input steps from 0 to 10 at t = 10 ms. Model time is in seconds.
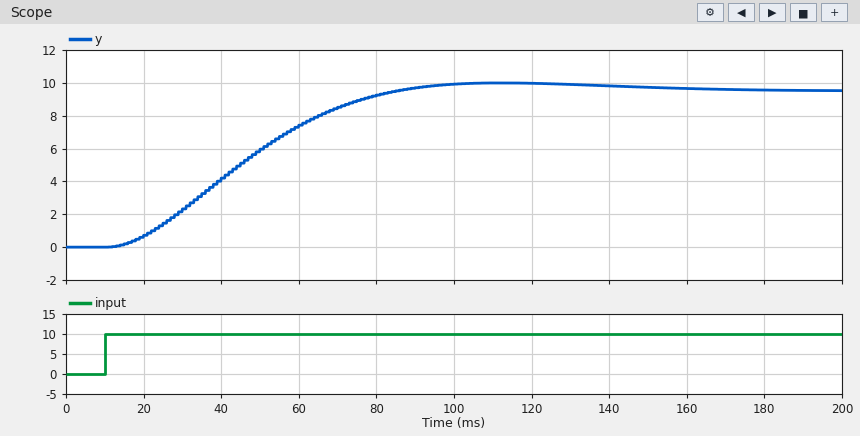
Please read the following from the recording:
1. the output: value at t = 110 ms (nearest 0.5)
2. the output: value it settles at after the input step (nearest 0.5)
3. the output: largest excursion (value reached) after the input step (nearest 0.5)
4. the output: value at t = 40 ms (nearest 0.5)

10.0
9.5
10.0
4.0
